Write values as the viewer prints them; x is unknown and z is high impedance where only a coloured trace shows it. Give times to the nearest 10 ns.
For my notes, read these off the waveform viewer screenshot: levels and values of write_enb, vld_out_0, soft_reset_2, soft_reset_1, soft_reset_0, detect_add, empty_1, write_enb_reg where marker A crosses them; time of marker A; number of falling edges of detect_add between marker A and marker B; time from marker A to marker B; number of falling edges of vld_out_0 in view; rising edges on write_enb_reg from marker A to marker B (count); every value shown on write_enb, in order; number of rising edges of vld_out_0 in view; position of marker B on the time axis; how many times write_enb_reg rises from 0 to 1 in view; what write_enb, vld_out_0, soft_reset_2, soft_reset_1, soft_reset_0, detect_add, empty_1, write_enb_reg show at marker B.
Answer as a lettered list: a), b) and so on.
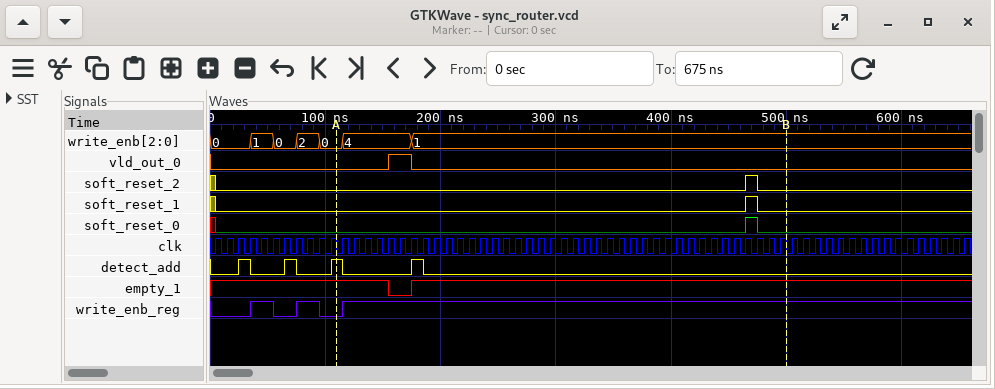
a) write_enb=0, vld_out_0=0, soft_reset_2=0, soft_reset_1=0, soft_reset_0=0, detect_add=1, empty_1=1, write_enb_reg=0
b) 110 ns
c) 2
d) 390 ns
e) 1
f) 1
g) 0, 1, 0, 2, 0, 4, 1
h) 1
i) 500 ns
j) 3
k) write_enb=1, vld_out_0=0, soft_reset_2=0, soft_reset_1=0, soft_reset_0=0, detect_add=0, empty_1=1, write_enb_reg=1
